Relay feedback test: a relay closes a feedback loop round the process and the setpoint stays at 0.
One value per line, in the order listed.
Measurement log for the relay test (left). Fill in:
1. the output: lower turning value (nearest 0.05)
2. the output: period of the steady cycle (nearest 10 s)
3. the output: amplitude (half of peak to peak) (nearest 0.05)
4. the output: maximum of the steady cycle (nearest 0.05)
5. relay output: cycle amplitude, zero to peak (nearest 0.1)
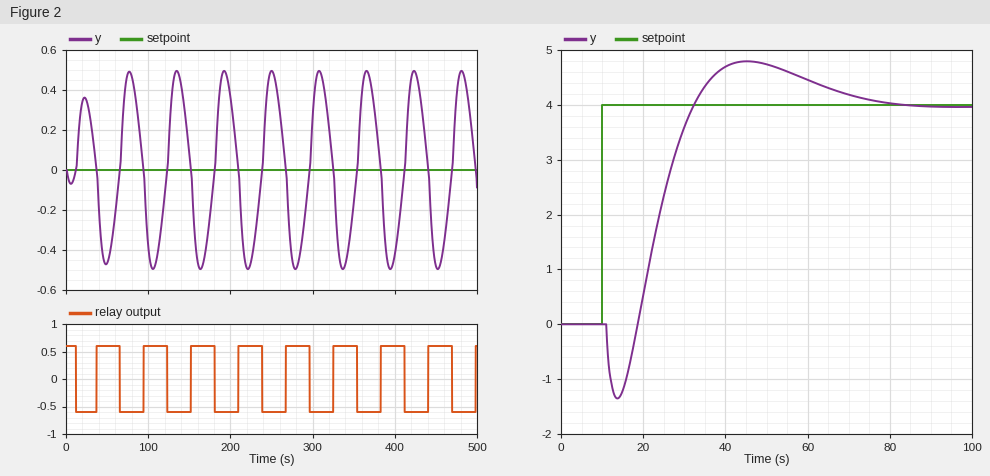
-0.50
60 s
0.50
0.50
0.6
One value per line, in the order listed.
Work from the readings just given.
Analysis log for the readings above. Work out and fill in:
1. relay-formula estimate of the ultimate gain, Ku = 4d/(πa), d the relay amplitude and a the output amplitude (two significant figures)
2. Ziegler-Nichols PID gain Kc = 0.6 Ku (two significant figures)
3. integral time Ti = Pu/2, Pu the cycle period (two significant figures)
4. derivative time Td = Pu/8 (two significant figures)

1.5
0.90
30 s
7.5 s
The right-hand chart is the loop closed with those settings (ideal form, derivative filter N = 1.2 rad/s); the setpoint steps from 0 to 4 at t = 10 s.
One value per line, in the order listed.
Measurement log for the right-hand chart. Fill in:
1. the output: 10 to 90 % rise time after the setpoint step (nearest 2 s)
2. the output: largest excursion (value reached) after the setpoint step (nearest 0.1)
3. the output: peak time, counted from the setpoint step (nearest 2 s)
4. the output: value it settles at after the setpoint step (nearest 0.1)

10 s
4.8
36 s
4.0
